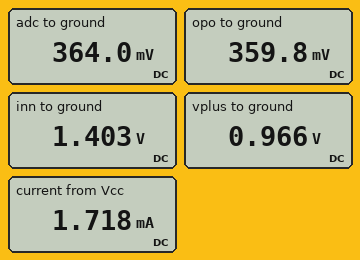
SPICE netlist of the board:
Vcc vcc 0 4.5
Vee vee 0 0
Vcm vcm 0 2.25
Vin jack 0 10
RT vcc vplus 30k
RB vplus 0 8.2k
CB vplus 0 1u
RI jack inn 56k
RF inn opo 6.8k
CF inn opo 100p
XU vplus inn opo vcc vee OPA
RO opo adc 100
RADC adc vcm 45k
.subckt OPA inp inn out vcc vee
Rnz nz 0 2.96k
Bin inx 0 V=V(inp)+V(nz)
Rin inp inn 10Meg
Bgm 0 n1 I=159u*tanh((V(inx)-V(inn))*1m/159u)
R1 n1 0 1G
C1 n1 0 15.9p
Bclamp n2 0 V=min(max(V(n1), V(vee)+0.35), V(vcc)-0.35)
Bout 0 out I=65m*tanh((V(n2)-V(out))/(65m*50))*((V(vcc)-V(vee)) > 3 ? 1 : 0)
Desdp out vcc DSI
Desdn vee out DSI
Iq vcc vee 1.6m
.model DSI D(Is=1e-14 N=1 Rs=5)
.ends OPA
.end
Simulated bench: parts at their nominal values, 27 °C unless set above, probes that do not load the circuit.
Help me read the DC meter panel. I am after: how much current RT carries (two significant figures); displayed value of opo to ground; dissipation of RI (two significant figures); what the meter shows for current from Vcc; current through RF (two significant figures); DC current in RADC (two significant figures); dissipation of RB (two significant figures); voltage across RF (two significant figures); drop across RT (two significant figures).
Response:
120 µA
359.8 mV
1.3 mW
1.718 mA
150 µA
42 µA
110 µW
1.0 V
3.5 V
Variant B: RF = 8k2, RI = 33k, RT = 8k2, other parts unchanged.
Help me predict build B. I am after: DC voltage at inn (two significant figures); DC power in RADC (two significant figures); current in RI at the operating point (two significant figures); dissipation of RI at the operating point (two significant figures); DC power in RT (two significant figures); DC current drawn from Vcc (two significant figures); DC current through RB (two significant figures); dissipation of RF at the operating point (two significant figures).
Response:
2.3 V
79 µW
230 µA
1.8 mW
620 µW
1.9 mA
270 µA
450 µW
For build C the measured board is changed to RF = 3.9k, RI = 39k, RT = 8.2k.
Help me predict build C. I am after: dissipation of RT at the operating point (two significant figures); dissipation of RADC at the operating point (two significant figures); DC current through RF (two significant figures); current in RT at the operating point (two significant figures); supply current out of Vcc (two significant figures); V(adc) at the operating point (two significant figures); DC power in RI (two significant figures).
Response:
620 µW
13 µW
200 µA
270 µA
1.9 mA
1.5 V
1.5 mW
